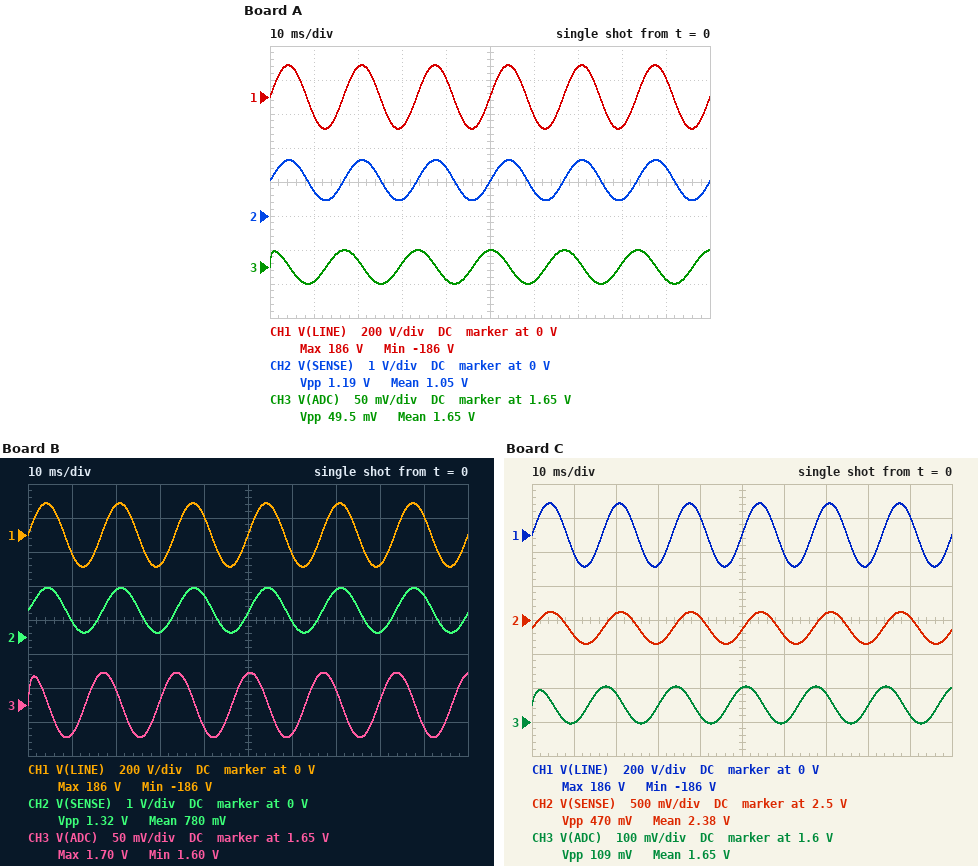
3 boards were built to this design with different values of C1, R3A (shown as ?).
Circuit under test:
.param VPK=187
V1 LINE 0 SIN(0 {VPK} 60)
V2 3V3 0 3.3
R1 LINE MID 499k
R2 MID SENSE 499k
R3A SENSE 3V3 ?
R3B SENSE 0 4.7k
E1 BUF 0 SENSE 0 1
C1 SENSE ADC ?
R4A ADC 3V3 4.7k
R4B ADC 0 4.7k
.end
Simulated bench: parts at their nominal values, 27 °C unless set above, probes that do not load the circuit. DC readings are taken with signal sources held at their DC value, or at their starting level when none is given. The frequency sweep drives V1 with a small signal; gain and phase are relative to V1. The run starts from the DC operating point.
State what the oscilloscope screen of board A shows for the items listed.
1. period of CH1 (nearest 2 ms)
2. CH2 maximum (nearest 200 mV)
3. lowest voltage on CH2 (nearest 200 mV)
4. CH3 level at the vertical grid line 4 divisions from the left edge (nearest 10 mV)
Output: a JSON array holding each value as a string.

["16 ms", "1.6 V", "400 mV", "1.63 V"]
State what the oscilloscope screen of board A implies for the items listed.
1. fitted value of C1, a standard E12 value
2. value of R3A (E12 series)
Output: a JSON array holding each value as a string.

["47 nF", "10 kΩ"]
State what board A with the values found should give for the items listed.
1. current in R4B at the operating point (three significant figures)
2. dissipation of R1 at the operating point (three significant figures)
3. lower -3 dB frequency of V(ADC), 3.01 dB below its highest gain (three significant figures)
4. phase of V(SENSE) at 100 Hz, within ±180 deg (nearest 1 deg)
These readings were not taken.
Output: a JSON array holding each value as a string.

["351 µA", "554 nW", "612 Hz", "-5 deg"]
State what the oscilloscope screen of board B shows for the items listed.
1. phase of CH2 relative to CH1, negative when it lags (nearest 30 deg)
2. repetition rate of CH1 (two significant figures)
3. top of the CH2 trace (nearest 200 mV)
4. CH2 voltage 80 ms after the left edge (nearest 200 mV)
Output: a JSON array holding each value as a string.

["0 deg", "60 Hz", "1.4 V", "200 mV"]
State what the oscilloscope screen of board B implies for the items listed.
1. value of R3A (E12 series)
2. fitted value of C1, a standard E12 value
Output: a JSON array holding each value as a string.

["15 kΩ", "82 nF"]
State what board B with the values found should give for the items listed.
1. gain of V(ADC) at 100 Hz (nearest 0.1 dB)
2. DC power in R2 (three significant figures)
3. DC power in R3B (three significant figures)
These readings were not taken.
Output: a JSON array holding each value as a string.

["-67.7 dB", "308 nW", "131 µW"]
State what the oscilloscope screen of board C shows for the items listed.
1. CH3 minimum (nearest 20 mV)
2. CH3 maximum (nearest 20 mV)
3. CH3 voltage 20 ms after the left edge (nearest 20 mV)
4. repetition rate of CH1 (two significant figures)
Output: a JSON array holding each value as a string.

["1.60 V", "1.70 V", "1.68 V", "60 Hz"]
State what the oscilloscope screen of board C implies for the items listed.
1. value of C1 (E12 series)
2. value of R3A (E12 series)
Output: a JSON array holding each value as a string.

["270 nF", "1.8 kΩ"]
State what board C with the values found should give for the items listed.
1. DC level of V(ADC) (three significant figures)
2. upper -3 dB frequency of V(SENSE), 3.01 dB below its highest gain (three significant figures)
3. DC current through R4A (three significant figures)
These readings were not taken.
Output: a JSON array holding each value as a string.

["1.65 V", "391 Hz", "351 µA"]
